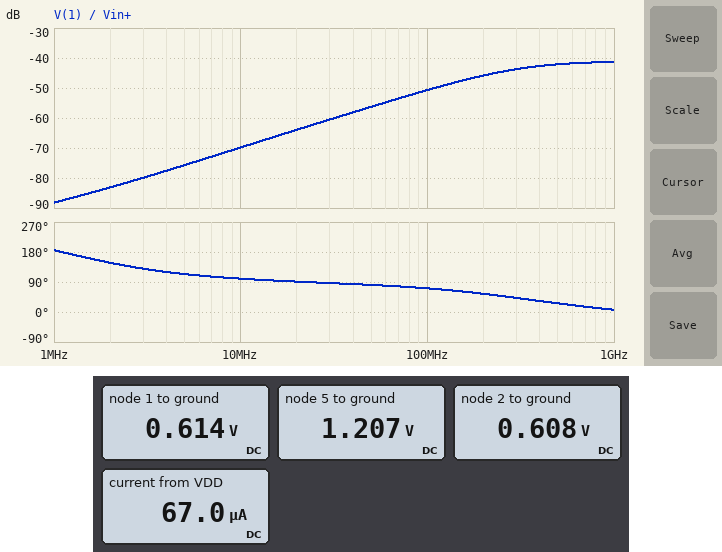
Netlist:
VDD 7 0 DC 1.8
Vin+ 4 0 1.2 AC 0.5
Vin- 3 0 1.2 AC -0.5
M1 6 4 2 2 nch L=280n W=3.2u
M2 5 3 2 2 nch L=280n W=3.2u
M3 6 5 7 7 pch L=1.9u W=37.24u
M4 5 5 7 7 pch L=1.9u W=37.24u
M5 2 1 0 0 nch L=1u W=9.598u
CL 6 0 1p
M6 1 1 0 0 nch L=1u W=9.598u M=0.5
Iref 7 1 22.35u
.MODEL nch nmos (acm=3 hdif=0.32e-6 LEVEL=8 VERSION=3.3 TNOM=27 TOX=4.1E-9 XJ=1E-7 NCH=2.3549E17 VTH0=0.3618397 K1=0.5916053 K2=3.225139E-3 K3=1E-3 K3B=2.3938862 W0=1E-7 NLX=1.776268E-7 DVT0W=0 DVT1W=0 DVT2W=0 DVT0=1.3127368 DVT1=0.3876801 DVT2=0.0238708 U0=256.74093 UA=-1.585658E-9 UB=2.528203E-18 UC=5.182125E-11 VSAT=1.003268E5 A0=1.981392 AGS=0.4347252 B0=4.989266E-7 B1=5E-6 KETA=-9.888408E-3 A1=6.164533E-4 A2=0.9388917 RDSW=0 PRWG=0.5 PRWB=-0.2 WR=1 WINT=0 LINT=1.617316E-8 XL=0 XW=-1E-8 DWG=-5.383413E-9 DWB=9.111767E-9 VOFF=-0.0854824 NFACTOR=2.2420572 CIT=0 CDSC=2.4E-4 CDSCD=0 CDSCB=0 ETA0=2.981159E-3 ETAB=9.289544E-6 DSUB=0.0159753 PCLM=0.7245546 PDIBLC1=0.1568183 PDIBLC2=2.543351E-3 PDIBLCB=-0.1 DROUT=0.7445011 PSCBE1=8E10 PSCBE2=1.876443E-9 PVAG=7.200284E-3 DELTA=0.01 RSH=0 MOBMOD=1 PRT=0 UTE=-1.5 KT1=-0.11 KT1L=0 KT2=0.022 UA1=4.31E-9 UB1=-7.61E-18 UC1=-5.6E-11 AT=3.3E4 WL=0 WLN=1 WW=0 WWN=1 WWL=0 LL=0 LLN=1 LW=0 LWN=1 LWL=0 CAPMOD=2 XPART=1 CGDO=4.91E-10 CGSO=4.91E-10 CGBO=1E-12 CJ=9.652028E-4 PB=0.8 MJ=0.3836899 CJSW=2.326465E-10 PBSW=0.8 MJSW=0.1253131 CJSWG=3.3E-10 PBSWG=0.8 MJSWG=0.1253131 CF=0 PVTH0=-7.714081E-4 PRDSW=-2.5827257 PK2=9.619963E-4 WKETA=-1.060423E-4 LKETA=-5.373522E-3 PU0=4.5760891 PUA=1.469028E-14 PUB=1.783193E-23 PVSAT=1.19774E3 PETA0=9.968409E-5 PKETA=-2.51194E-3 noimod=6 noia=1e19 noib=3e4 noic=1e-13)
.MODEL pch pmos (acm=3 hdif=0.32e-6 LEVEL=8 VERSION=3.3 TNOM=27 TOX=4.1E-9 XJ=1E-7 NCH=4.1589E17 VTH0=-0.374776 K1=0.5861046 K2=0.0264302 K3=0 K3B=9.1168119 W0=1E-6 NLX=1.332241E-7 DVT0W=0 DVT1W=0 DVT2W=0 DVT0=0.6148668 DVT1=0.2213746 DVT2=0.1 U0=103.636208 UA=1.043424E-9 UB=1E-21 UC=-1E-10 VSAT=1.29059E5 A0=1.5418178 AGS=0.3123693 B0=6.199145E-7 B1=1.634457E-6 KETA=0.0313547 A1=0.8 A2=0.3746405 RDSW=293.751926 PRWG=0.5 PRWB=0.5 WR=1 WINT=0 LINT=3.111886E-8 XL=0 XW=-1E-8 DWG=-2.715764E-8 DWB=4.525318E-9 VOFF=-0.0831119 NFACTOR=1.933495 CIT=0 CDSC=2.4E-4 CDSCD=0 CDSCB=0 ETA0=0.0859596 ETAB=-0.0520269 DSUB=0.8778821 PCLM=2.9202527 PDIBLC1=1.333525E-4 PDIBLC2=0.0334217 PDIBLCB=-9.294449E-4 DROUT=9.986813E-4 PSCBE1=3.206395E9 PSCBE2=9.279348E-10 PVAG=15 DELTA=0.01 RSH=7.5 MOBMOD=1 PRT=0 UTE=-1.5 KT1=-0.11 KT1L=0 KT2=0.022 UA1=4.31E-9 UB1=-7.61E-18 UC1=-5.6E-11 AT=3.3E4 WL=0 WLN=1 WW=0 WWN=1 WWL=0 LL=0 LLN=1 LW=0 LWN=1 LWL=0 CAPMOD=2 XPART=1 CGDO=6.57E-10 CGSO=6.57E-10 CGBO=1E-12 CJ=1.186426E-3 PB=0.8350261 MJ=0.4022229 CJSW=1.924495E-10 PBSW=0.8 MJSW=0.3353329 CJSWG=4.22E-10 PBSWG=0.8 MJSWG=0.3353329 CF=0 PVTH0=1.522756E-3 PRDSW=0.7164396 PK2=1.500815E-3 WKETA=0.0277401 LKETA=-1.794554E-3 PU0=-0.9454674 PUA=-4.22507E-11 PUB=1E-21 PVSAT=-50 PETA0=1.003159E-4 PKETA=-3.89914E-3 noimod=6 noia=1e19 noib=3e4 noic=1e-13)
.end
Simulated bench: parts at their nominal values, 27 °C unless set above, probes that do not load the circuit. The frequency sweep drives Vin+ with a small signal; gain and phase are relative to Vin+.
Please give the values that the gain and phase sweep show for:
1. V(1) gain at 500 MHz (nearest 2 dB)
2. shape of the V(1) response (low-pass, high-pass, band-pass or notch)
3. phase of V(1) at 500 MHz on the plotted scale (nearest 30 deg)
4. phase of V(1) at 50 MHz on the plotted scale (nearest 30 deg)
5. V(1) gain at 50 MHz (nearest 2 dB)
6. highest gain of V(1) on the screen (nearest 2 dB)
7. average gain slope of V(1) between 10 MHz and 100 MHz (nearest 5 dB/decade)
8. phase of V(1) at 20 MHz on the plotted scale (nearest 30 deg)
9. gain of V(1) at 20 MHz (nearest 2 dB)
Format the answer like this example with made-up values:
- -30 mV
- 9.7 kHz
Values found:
- -42 dB
- high-pass
- 30 deg
- 90 deg
- -56 dB
- -42 dB
- 20 dB/decade
- 90 deg
- -64 dB
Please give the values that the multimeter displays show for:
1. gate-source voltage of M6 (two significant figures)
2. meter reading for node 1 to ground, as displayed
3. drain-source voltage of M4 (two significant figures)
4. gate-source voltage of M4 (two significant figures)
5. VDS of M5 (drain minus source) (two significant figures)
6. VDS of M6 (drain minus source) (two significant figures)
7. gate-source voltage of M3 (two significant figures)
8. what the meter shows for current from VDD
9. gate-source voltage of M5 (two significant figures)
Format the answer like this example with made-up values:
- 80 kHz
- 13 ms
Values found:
- 610 mV
- 0.614 V
- -590 mV
- -590 mV
- 610 mV
- 610 mV
- -590 mV
- 67.0 µA
- 610 mV
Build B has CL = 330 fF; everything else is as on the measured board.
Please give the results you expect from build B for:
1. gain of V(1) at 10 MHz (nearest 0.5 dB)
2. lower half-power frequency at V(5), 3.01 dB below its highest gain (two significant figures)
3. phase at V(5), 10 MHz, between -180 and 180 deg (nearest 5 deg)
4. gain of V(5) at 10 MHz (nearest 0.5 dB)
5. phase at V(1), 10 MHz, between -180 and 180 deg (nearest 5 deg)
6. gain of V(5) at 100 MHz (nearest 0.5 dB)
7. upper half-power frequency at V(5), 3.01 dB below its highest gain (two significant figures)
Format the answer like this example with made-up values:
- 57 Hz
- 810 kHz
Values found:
- -69.5 dB
- 2.1 MHz
- -5 deg
- -0.5 dB
- 120 deg
- -9.5 dB
- 40 MHz
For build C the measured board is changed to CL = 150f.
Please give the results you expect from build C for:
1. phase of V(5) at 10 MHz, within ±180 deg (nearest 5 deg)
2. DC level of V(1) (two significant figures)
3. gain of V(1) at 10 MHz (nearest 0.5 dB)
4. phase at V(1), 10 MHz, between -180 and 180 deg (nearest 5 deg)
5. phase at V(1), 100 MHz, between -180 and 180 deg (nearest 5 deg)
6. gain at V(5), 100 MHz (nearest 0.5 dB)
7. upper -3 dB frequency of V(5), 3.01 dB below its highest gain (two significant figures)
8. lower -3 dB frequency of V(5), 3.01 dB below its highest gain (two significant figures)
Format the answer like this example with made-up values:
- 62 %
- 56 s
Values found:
- 5 deg
- 610 mV
- -69.0 dB
- 140 deg
- 75 deg
- -10.0 dB
- 45 MHz
- 3.4 MHz
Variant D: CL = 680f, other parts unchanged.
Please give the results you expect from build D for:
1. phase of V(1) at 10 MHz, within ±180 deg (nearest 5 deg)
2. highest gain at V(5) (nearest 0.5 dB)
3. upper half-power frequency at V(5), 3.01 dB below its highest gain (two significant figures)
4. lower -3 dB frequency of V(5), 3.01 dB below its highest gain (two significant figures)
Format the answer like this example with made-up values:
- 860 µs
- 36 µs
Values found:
- 105 deg
- 0 dB
- 38 MHz
- 1.2 MHz
